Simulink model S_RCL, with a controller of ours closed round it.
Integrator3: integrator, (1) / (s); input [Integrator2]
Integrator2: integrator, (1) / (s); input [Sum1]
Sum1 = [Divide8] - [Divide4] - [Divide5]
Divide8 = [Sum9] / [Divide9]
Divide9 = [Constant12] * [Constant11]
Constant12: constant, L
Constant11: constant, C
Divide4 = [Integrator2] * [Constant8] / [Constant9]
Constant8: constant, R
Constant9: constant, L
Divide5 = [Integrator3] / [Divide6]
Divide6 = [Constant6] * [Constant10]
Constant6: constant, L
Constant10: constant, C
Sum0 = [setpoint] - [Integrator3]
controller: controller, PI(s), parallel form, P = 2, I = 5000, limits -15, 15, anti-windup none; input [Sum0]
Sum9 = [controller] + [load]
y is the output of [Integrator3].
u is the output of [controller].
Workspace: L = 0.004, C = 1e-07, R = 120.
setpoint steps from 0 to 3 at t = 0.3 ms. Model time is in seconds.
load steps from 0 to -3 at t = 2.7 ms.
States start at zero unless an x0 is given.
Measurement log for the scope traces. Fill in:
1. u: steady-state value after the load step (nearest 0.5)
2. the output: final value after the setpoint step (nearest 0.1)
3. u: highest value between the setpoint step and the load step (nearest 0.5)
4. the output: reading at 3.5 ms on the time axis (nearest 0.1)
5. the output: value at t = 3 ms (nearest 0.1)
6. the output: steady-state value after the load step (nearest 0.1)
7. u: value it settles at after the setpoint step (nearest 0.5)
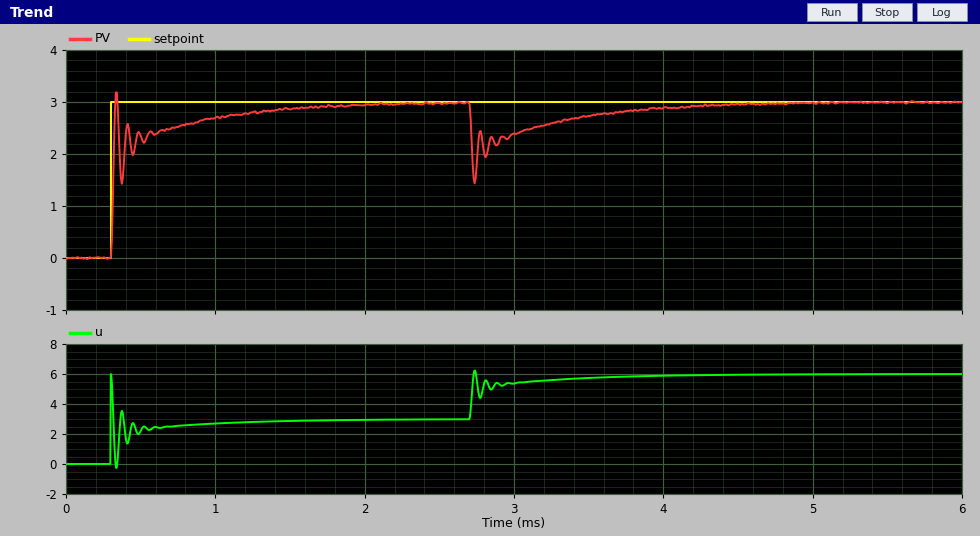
6.0
3.0
6.0
2.7
2.4
3.0
3.0
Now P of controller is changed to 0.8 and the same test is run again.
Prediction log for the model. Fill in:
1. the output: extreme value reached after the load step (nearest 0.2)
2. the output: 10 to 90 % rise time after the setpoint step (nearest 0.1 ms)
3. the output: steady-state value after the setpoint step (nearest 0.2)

0.6
0.6 ms
3.0
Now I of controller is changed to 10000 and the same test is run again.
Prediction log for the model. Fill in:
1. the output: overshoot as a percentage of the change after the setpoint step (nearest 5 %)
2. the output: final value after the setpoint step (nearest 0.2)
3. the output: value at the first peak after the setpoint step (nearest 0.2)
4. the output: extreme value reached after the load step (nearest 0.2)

10 %
3.0
3.4
1.4
